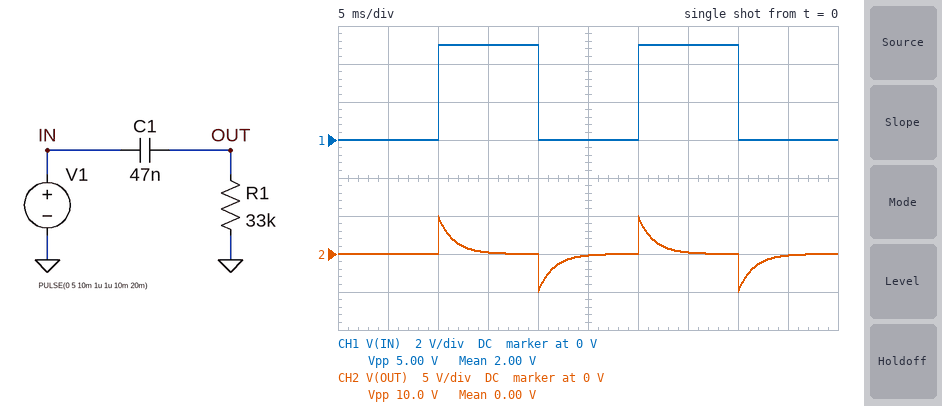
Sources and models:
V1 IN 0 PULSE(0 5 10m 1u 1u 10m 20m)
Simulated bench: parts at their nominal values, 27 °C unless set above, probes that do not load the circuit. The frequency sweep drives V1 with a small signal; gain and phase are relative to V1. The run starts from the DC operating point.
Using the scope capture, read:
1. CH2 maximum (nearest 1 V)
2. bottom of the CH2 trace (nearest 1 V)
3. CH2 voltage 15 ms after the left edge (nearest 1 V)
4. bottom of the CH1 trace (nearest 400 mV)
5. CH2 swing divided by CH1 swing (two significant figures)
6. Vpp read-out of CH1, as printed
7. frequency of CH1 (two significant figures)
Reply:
5 V
-5 V
0 V
0 V
2.0
5.00 V
50 Hz
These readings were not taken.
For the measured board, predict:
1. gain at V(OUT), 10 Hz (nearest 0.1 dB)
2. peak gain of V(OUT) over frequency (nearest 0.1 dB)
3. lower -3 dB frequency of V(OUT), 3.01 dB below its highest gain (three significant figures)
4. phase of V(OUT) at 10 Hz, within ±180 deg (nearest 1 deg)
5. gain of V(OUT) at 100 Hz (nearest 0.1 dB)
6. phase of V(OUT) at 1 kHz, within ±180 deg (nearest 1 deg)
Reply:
-20.3 dB
0 dB
103 Hz
84 deg
-3.1 dB
6 deg
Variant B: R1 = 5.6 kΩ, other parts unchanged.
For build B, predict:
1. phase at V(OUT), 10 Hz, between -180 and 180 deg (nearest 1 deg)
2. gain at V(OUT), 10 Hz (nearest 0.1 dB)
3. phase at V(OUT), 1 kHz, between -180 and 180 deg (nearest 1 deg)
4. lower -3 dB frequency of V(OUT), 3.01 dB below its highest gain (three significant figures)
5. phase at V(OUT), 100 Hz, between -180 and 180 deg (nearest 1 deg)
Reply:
89 deg
-35.6 dB
31 deg
605 Hz
81 deg
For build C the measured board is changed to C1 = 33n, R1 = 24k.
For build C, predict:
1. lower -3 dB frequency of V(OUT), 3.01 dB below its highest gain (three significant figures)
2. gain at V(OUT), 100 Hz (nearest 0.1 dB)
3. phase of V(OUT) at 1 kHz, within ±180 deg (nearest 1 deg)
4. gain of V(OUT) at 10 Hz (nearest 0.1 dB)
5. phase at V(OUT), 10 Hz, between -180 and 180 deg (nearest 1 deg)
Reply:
201 Hz
-7.0 dB
11 deg
-26.1 dB
87 deg
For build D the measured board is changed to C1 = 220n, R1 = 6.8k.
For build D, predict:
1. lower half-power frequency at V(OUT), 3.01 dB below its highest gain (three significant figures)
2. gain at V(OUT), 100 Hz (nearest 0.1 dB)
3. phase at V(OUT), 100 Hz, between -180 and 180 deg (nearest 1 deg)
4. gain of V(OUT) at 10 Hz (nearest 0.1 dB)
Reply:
106 Hz
-3.3 dB
47 deg
-20.6 dB
